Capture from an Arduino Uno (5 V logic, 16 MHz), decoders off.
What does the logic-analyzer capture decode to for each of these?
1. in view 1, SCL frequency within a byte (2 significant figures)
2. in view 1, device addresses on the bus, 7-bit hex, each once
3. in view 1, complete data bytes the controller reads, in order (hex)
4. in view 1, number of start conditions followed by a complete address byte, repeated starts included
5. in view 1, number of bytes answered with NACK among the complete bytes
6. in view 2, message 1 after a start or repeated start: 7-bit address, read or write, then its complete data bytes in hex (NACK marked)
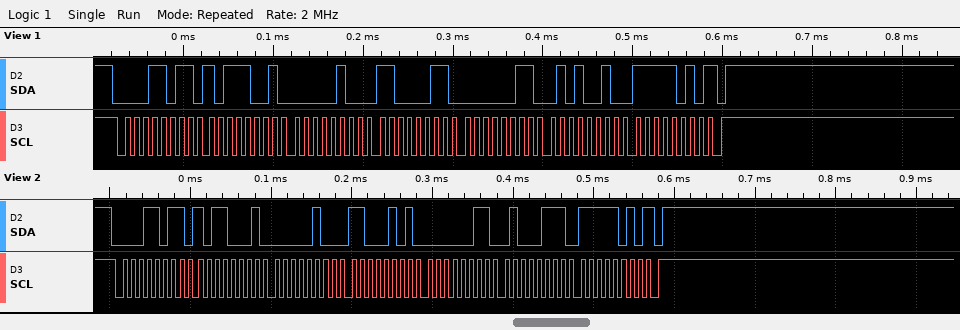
100 kHz
0x0D
B9 04 C3 03 52 FA
1
1
0x0D read: B1 04 C5 03 47 FA NACK
